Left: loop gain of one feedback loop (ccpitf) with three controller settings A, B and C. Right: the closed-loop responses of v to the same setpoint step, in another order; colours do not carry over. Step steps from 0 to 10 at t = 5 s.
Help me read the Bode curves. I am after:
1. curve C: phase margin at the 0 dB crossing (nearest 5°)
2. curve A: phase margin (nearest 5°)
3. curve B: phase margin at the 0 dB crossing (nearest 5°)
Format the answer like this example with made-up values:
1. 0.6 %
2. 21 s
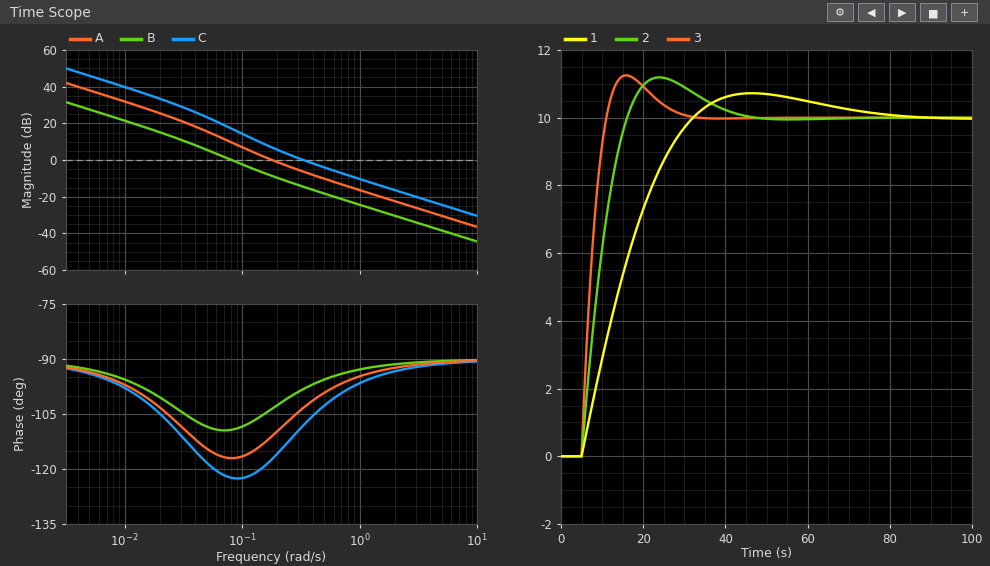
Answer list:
1. 70°
2. 70°
3. 70°
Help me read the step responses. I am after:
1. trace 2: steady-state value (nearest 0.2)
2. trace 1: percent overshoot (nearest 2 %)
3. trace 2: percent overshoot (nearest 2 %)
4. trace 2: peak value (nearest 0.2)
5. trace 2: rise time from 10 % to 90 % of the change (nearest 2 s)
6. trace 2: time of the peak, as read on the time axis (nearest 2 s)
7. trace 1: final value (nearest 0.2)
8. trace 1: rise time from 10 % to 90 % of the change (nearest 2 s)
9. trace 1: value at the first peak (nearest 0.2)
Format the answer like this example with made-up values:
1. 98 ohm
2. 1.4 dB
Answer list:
1. 10.0
2. 8 %
3. 12 %
4. 11.2
5. 8 s
6. 24 s
7. 10.0
8. 20 s
9. 10.8
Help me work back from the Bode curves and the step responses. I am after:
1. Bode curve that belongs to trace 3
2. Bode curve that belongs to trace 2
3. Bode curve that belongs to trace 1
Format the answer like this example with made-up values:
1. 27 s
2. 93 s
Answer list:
1. C
2. A
3. B
